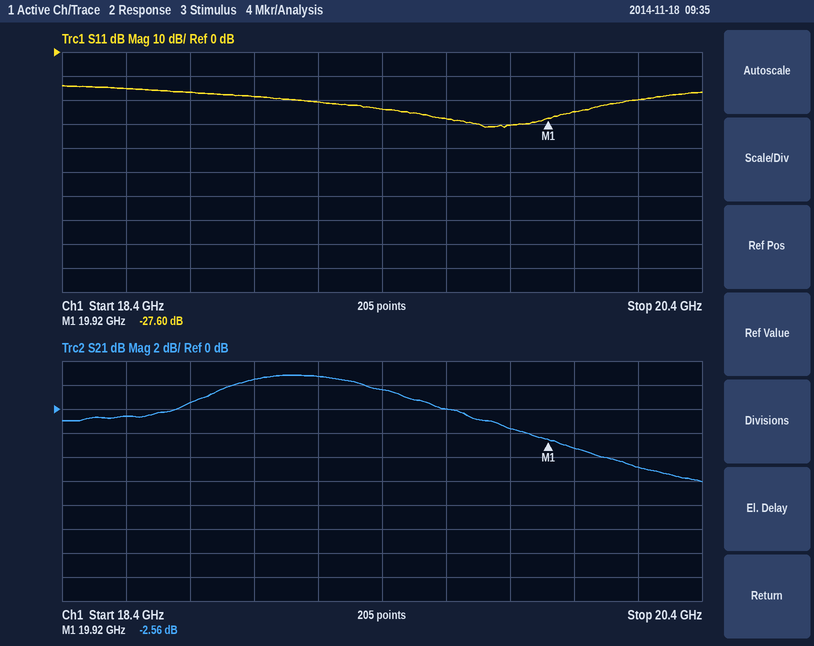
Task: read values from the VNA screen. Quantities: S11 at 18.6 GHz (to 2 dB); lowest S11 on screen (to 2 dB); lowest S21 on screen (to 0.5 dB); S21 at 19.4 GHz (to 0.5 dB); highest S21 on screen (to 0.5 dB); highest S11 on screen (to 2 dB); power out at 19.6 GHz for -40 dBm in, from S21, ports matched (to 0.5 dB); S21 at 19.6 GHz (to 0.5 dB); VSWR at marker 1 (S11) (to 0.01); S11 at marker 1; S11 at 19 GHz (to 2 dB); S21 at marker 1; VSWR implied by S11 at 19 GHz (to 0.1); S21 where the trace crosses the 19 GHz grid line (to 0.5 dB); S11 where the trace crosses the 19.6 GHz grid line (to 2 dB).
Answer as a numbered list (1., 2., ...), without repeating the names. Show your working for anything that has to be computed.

1. -16 dB
2. -32 dB
3. -6.0 dB
4. 1.5 dB
5. 3.0 dB
6. -14 dB
7. -40 dBm + (0.0 dB) = -40.0 dBm
8. 0.0 dB
9. (1 + 0.0417)/(1 − 0.0417) ≈ 1.09
10. -27.60 dB
11. -18 dB
12. -2.56 dB
13. |Γ| = 10^(-18/20) = 0.1259; VSWR = (1 + 0.1259)/(1 − 0.1259) ≈ 1.3
14. 2.5 dB
15. -28 dB
